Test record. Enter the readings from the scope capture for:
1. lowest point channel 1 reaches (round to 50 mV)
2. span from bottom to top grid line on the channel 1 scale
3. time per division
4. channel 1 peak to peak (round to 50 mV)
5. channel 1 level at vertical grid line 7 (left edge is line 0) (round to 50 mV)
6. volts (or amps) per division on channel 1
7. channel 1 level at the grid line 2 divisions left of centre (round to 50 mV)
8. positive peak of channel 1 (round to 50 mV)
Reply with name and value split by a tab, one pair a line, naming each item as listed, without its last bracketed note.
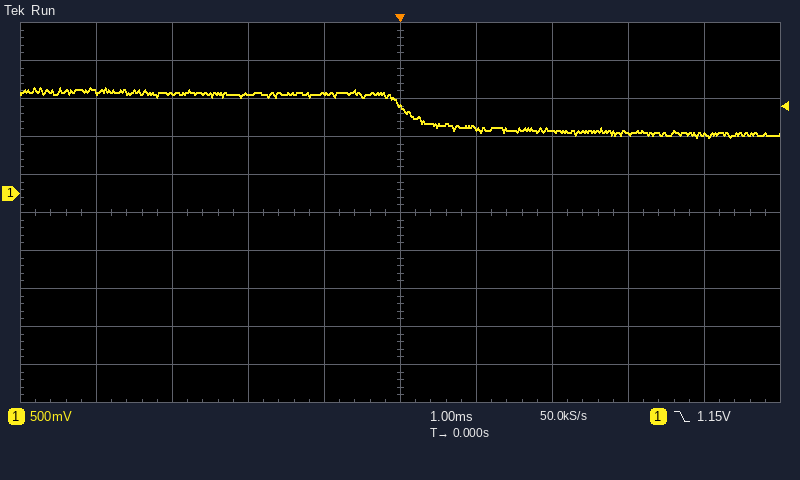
lowest point channel 1 reaches	750 mV
span from bottom to top grid line on the channel 1 scale	5 V
time per division	1 ms
channel 1 peak to peak	650 mV
channel 1 level at vertical grid line 7 (left edge is line 0)	800 mV
volts (or amps) per division on channel 1	500 mV
channel 1 level at the grid line 2 divisions left of centre	1.30 V
positive peak of channel 1	1.40 V
